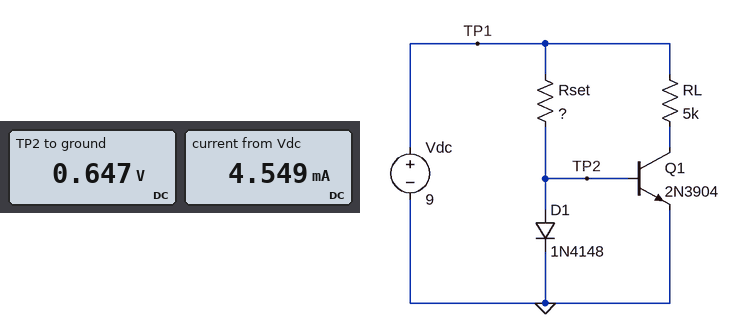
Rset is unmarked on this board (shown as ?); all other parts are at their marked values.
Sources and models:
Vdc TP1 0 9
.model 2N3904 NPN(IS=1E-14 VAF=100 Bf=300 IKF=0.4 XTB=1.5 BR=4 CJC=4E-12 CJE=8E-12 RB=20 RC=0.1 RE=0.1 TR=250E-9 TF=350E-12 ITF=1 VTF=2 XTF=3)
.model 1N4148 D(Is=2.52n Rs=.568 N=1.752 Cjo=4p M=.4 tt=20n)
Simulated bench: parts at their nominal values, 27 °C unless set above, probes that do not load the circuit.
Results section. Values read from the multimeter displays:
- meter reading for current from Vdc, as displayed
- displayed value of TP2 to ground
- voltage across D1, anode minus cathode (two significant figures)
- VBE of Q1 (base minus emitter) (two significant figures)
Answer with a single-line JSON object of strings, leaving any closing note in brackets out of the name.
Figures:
{"meter reading for current from Vdc, as displayed": "4.549 mA", "displayed value of TP2 to ground": "0.647 V", "voltage across D1, anode minus cathode": "650 mV", "VBE of Q1 (base minus emitter)": "650 mV"}
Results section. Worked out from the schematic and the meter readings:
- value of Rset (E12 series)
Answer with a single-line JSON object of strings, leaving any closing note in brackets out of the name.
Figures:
{"value of Rset": "2.2 kΩ"}
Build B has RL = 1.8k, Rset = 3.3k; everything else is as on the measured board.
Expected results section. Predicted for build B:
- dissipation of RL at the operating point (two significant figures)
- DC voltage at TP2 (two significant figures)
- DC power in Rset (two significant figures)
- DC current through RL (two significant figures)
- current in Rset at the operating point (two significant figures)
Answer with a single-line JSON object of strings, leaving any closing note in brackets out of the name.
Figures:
{"dissipation of RL at the operating point": "250 µW", "DC voltage at TP2": "630 mV", "DC power in Rset": "21 mW", "DC current through RL": "370 µA", "current in Rset at the operating point": "2.5 mA"}
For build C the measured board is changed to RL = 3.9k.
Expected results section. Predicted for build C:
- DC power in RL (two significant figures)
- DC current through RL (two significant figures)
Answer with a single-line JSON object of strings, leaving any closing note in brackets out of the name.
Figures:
{"DC power in RL": "2.2 mW", "DC current through RL": "760 µA"}
